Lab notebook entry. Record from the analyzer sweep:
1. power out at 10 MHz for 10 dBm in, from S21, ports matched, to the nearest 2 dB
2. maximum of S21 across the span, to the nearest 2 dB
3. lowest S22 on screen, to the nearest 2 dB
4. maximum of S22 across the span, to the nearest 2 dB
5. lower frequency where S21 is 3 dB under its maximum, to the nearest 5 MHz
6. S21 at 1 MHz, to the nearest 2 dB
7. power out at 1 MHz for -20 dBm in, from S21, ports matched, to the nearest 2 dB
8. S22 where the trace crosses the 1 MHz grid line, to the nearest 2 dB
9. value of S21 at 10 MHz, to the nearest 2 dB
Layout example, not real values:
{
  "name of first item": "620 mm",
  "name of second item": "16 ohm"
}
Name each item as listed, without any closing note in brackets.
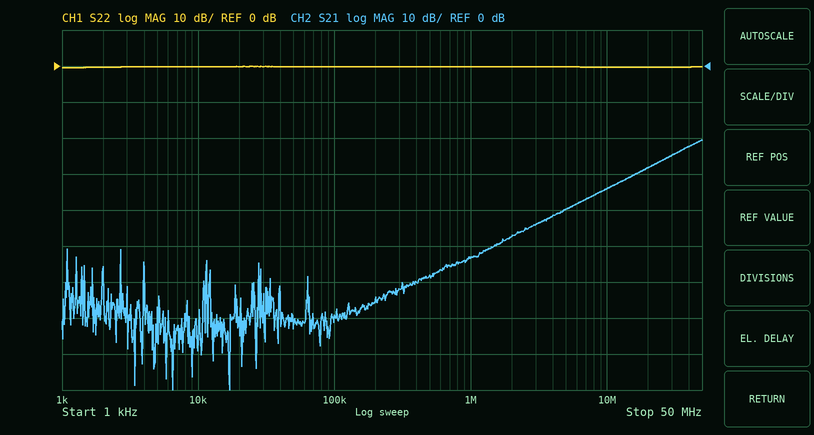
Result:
{
  "power out at 10 MHz for 10 dBm in, from S21, ports matched, to the nearest 2 dB": "-24 dBm",
  "maximum of S21 across the span, to the nearest 2 dB": "-20 dB",
  "lowest S22 on screen, to the nearest 2 dB": "0 dB",
  "maximum of S22 across the span, to the nearest 2 dB": "0 dB",
  "lower frequency where S21 is 3 dB under its maximum, to the nearest 5 MHz": "35 MHz",
  "S21 at 1 MHz, to the nearest 2 dB": "-54 dB",
  "power out at 1 MHz for -20 dBm in, from S21, ports matched, to the nearest 2 dB": "-74 dBm",
  "S22 where the trace crosses the 1 MHz grid line, to the nearest 2 dB": "0 dB",
  "value of S21 at 10 MHz, to the nearest 2 dB": "-34 dB"
}
